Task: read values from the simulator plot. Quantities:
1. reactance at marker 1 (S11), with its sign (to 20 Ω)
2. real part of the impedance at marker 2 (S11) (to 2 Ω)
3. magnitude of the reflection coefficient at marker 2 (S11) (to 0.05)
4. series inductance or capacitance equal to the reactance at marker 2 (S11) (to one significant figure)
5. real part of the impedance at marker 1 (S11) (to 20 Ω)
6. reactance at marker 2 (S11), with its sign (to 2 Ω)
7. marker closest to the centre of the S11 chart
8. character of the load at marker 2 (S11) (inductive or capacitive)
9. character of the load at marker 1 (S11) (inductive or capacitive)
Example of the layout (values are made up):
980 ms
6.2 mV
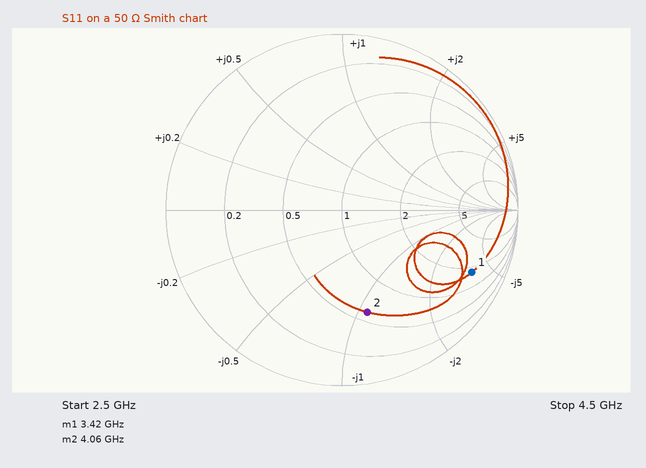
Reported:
-180 Ω
30 Ω
0.60
700 fF
80 Ω
-54 Ω
marker 2
capacitive
capacitive
